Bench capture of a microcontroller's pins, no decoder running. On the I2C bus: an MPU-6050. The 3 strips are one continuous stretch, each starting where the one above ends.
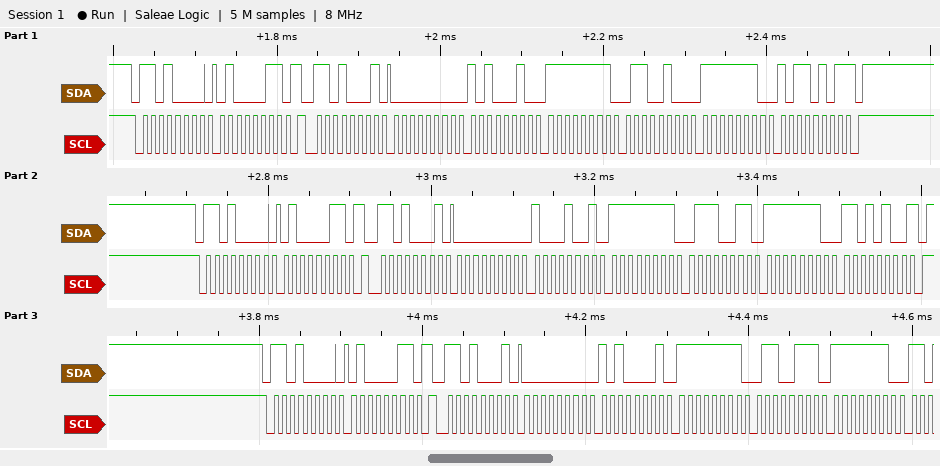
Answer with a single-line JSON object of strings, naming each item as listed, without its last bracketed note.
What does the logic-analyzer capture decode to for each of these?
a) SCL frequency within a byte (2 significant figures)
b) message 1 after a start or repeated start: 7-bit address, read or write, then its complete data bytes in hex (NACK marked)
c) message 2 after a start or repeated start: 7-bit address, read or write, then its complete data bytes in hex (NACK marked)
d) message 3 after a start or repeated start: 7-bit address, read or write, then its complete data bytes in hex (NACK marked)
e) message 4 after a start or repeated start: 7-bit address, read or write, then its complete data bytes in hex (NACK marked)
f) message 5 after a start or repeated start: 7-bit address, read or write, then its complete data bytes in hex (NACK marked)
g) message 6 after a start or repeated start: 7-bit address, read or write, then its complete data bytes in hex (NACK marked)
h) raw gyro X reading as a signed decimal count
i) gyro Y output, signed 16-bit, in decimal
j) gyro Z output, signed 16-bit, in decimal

{"SCL frequency within a byte": "100 kHz", "message 1 after a start or repeated start: 7-bit address, read or write, then its complete data bytes in hex": "0x68 write: 43", "message 2 after a start or repeated start: 7-bit address, read or write, then its complete data bytes in hex": "0x68 read: 00 A2 FF 64 FE B5 NACK", "message 3 after a start or repeated start: 7-bit address, read or write, then its complete data bytes in hex": "0x68 write: 43", "message 4 after a start or repeated start: 7-bit address, read or write, then its complete data bytes in hex": "0x68 read: 00 89 FF 73 FE D4 NACK", "message 5 after a start or repeated start: 7-bit address, read or write, then its complete data bytes in hex": "0x68 write: 43", "message 6 after a start or repeated start: 7-bit address, read or write, then its complete data bytes in hex": "0x68 read: 00 A1 FF 67 FE", "raw gyro X reading as a signed decimal count": "162", "gyro Y output, signed 16-bit, in decimal": "-156", "gyro Z output, signed 16-bit, in decimal": "-331"}
